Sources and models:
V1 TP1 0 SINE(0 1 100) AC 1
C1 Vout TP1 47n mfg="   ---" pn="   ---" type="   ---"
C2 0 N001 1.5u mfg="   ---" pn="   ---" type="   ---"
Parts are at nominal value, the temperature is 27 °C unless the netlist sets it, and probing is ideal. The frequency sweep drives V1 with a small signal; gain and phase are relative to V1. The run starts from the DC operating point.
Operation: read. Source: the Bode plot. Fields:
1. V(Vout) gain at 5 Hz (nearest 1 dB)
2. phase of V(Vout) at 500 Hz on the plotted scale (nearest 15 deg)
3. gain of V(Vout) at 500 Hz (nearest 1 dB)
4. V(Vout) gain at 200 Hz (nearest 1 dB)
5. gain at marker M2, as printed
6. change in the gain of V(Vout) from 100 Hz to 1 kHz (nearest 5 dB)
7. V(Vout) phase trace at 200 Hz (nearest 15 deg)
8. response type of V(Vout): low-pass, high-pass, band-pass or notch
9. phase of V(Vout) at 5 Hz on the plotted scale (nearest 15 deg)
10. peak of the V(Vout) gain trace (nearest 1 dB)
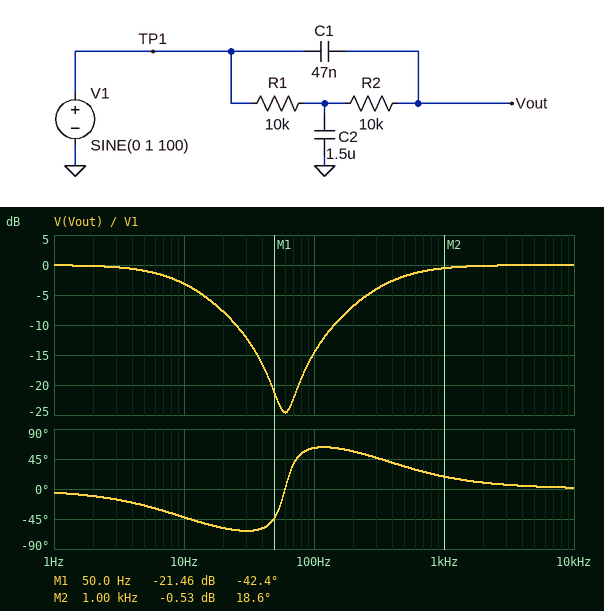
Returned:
-1 dB
30 deg
-2 dB
-7 dB
-0.53 dB
15 dB
60 deg
notch
-30 deg
0 dB
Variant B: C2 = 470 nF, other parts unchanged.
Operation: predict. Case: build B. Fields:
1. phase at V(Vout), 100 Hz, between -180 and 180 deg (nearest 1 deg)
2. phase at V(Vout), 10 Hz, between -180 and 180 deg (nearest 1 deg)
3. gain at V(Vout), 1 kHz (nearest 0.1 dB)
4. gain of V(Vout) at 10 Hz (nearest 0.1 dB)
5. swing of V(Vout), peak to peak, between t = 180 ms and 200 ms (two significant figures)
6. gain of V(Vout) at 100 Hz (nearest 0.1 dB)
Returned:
-10 deg
-16 deg
-0.7 dB
-0.5 dB
340 mV
-15.4 dB
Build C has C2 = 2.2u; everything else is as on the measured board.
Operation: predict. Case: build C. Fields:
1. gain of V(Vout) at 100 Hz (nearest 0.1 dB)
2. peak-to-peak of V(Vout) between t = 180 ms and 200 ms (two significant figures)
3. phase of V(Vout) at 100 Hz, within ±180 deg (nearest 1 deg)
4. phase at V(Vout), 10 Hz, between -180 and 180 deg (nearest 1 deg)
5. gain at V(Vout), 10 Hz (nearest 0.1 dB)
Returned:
-13.4 dB
430 mV
67 deg
-53 deg
-5.1 dB
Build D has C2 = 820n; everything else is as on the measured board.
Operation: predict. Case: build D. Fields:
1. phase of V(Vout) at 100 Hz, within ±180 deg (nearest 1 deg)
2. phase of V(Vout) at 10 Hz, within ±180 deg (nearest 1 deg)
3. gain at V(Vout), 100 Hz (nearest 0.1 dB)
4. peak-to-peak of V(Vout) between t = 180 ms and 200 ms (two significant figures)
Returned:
36 deg
-27 deg
-17.3 dB
270 mV
